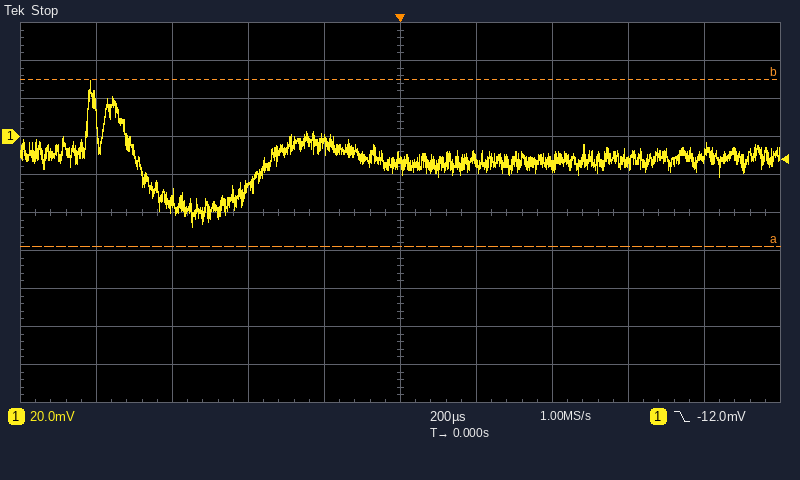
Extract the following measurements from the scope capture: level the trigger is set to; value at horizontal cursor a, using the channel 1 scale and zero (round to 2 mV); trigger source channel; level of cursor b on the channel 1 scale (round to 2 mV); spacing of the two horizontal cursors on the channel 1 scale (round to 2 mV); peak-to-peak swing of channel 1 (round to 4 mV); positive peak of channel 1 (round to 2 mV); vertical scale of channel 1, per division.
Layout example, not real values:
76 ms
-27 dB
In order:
-12.0 mV
-58 mV
channel 1
30 mV
88 mV
76 mV
30 mV
20 mV
